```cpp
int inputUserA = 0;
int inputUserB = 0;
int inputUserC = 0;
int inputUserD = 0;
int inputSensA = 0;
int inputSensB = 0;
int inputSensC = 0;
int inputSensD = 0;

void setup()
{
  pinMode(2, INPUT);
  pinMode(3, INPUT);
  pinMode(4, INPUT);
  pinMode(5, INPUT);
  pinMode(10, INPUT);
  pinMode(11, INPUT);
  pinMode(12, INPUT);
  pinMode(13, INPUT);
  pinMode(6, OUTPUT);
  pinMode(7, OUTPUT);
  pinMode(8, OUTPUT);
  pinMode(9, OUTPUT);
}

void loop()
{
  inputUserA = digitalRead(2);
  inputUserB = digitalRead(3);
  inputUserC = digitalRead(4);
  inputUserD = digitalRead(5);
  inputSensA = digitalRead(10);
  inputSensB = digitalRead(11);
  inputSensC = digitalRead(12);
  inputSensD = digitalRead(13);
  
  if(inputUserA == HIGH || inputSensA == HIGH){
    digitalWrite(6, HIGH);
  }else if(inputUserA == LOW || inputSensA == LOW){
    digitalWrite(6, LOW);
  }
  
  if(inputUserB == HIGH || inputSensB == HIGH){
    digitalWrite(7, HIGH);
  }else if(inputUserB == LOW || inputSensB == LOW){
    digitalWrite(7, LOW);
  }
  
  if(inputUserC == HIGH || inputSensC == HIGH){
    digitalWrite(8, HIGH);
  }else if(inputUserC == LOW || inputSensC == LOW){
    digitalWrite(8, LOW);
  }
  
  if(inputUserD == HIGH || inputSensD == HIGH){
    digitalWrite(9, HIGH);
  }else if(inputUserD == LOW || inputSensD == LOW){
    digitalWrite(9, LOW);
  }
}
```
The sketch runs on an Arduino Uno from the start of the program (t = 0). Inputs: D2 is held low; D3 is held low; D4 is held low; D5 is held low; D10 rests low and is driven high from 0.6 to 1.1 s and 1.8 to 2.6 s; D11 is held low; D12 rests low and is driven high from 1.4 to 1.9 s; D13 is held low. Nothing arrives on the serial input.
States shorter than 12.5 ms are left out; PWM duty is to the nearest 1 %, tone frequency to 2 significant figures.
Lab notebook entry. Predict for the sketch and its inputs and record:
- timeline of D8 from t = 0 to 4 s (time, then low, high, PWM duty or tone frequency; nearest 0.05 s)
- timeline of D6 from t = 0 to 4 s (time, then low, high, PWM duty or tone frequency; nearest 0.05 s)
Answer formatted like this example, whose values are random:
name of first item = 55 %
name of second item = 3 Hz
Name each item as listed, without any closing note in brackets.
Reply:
timeline of D8 from t = 0 to 4 s = 0 s low; 1.4 s high; 1.9 s low
timeline of D6 from t = 0 to 4 s = 0 s low; 0.6 s high; 1.1 s low; 1.8 s high; 2.6 s low
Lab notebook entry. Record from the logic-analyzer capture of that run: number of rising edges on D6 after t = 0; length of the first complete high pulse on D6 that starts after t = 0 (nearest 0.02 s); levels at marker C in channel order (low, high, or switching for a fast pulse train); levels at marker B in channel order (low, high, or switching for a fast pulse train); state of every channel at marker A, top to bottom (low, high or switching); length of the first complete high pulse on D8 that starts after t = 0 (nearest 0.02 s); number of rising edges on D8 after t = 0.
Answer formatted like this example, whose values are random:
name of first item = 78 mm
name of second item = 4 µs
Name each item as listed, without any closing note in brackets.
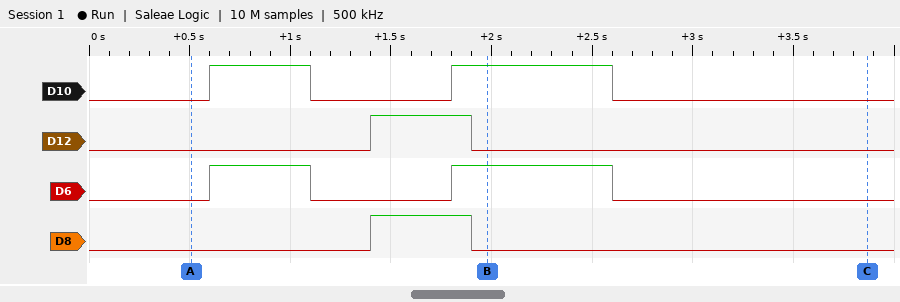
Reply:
number of rising edges on D6 after t = 0 = 2
length of the first complete high pulse on D6 that starts after t = 0 = 0.50 s
levels at marker C in channel order = D10 low, D12 low, D6 low, D8 low
levels at marker B in channel order = D10 high, D12 low, D6 high, D8 low
state of every channel at marker A, top to bottom = D10 low, D12 low, D6 low, D8 low
length of the first complete high pulse on D8 that starts after t = 0 = 0.50 s
number of rising edges on D8 after t = 0 = 1
